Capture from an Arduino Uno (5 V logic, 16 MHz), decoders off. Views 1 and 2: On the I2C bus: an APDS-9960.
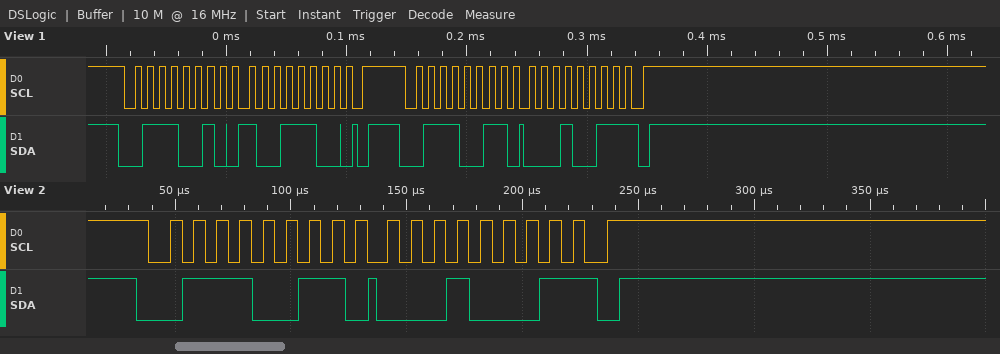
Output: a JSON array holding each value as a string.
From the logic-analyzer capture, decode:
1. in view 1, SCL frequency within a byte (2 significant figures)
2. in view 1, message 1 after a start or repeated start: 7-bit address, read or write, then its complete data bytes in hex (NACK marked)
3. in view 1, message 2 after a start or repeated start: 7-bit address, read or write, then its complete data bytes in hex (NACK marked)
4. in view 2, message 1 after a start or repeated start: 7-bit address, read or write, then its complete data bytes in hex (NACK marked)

["100 kHz", "0x39 write: 9C", "0x39 read: 13 NACK", "0x39 read: 11 NACK"]
